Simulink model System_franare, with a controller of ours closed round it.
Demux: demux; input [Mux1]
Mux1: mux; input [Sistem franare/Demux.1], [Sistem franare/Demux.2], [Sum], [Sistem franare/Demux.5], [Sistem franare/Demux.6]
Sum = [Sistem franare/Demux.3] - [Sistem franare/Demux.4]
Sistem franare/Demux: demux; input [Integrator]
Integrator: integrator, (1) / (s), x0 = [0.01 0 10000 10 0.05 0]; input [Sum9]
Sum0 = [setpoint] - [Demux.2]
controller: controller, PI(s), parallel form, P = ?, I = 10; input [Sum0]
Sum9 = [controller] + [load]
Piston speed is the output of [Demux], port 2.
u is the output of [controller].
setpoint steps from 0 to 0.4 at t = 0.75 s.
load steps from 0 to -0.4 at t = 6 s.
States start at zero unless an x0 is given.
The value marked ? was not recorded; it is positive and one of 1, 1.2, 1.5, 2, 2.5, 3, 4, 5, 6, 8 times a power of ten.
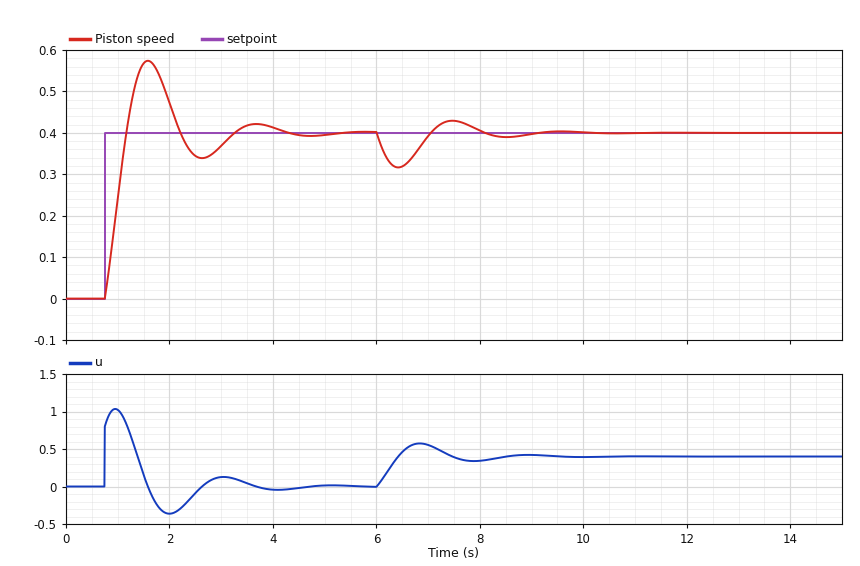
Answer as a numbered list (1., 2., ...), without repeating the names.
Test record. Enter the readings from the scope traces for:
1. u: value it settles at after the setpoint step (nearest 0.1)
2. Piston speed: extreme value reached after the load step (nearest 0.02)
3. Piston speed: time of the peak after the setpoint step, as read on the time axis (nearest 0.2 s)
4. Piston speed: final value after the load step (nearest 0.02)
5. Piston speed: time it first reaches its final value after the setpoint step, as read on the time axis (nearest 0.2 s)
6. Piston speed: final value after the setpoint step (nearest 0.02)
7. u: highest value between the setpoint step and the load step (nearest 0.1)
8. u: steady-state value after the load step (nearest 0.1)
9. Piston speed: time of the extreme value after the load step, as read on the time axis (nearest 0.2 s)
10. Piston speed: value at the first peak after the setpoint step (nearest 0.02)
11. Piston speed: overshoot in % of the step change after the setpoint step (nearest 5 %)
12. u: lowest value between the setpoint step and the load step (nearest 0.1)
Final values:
1. 0.0
2. 0.32
3. 1.6 s
4. 0.40
5. 1.2 s
6. 0.40
7. 1.0
8. 0.4
9. 6.4 s
10. 0.58
11. 45 %
12. -0.4
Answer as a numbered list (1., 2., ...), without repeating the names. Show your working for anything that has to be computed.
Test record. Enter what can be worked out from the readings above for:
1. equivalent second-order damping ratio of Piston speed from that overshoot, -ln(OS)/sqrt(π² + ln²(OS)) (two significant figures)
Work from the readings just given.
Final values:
1. ln(0.45) = -0.799; 0.799 / sqrt(9.870 + 0.638) = 0.25
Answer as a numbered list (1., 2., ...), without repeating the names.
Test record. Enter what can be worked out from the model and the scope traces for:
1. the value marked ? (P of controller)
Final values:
1. 2
